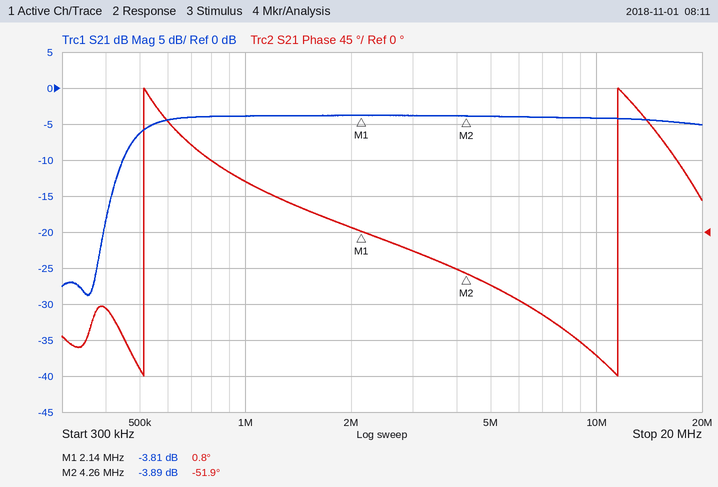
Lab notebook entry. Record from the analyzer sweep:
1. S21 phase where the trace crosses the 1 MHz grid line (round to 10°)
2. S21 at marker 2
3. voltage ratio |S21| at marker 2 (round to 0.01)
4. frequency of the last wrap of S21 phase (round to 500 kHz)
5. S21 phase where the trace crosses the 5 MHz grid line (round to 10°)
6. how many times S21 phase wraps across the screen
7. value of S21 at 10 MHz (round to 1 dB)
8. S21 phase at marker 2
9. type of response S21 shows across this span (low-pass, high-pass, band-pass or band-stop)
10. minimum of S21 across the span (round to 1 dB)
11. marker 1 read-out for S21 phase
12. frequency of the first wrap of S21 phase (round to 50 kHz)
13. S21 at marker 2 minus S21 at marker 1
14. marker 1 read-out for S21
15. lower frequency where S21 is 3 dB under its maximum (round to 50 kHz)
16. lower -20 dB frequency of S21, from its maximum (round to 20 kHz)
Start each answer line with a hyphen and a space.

- 60°
- -3.89 dB
- 0.64
- 11.5 MHz
- -70°
- 2
- -4 dB
- -51.9°
- high-pass
- -29 dB
- 0.8°
- 500 kHz
- -0.08 dB
- -3.81 dB
- 500 kHz
- 380 kHz
